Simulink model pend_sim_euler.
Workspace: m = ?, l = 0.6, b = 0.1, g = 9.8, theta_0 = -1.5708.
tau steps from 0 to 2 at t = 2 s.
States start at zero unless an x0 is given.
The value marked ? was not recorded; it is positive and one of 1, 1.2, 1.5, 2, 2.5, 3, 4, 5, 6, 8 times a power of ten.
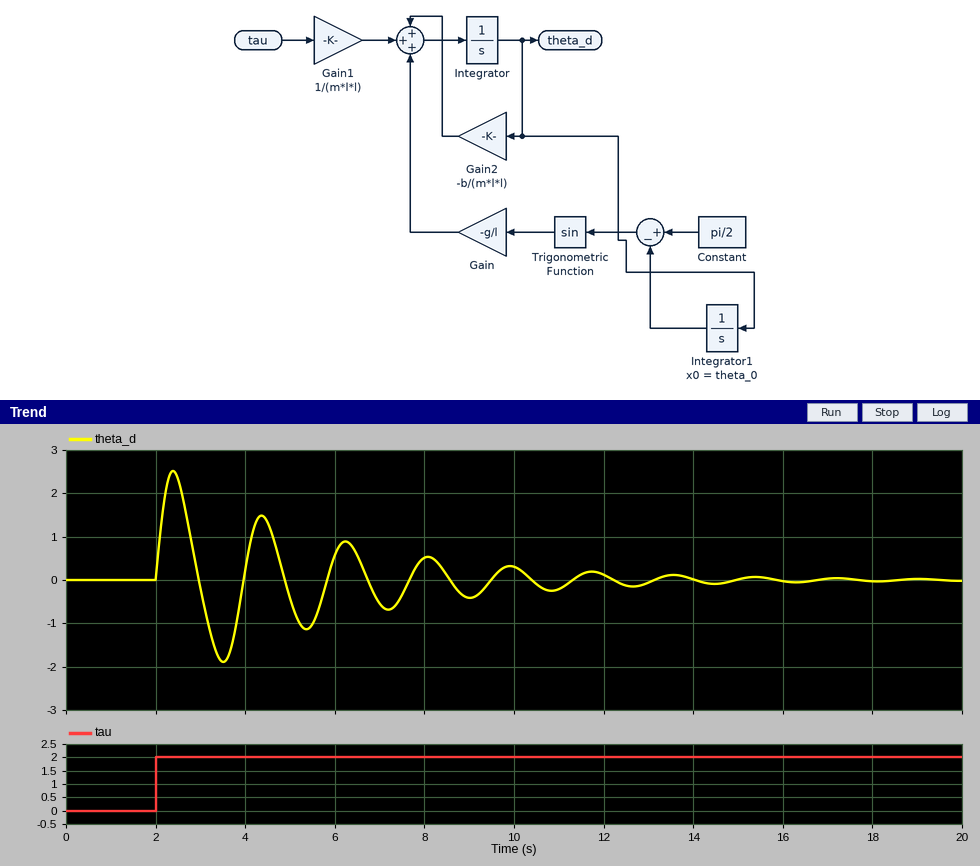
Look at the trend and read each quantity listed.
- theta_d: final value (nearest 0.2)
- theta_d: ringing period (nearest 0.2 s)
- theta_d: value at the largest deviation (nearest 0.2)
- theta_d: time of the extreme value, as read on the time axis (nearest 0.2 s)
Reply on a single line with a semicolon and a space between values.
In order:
0.0; 2.0 s; 2.6; 2.4 s
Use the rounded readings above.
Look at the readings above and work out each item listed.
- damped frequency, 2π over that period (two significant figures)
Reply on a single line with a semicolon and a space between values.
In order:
3.1 rad/s
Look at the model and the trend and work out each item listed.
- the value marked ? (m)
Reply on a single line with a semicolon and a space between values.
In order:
0.5
